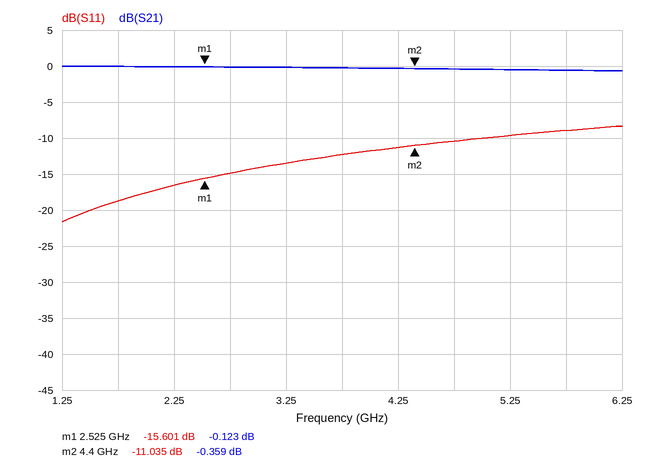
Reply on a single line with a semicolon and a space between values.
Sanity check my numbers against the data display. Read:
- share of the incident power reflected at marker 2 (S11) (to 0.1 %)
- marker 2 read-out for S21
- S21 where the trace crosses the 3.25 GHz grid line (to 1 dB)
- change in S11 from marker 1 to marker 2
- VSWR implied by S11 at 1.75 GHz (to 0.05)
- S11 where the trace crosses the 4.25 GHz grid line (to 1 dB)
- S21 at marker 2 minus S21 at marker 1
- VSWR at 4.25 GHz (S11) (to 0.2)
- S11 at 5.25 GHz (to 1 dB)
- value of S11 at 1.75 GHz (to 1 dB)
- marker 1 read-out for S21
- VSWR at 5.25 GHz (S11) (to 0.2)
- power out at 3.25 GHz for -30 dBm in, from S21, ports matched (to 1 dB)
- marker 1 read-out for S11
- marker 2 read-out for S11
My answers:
7.9 %; -0.359 dB; 0 dB; 4.566 dB; 1.25; -11 dB; -0.236 dB; 1.8; -10 dB; -19 dB; -0.123 dB; 2.0; -30 dBm; -15.601 dB; -11.035 dB
